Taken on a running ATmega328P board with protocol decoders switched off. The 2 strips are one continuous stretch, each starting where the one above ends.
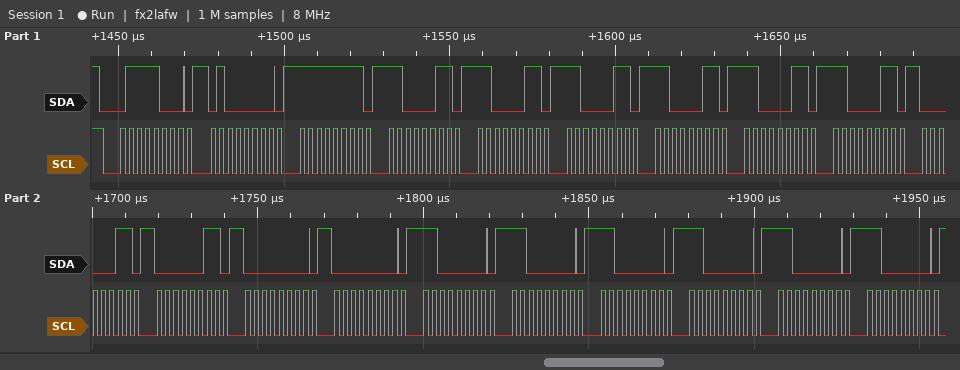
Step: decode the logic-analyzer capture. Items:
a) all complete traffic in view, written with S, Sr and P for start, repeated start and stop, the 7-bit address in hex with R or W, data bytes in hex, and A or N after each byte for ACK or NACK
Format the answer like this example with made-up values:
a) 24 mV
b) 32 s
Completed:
a) S 3CW A 40 A FF A C3 A C3 A C3 A C3 A C3 A C3 A 03 A 03 A 00 A 00 A C0 A C0 A C0 A C0 A C0 A C0 A
